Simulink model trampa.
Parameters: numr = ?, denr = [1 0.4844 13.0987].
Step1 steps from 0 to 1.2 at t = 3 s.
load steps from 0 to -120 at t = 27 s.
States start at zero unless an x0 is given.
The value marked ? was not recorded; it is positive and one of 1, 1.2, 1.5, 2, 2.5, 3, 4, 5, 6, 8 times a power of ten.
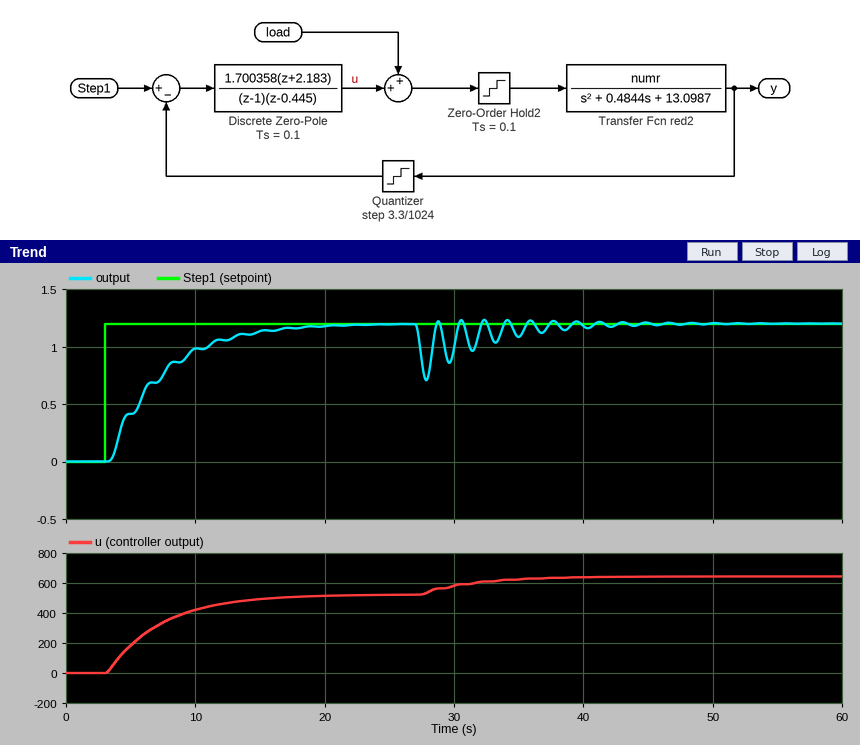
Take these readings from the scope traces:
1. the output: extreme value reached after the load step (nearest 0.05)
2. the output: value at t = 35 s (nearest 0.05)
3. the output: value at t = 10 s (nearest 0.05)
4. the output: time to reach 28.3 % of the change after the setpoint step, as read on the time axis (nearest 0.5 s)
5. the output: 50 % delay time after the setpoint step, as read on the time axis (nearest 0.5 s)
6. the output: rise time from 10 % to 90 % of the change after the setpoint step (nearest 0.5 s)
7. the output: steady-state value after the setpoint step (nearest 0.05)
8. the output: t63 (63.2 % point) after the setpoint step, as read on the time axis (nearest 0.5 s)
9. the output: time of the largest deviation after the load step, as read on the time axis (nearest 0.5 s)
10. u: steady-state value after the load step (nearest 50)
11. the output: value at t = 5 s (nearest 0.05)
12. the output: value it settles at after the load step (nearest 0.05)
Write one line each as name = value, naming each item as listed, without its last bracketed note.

the output: extreme value reached after the load step = 0.70
the output: value at t = 35 s = 1.10
the output: value at t = 10 s = 1.00
the output: time to reach 28.3 % of the change after the setpoint step, as read on the time axis = 4.5 s
the output: 50 % delay time after the setpoint step, as read on the time axis = 6.0 s
the output: rise time from 10 % to 90 % of the change after the setpoint step = 9.0 s
the output: steady-state value after the setpoint step = 1.20
the output: t63 (63.2 % point) after the setpoint step, as read on the time axis = 7.5 s
the output: time of the largest deviation after the load step, as read on the time axis = 28.0 s
u: steady-state value after the load step = 650
the output: value at t = 5 s = 0.40
the output: value it settles at after the load step = 1.20
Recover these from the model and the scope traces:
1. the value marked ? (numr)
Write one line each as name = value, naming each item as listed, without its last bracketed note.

the value marked ? = 0.03
